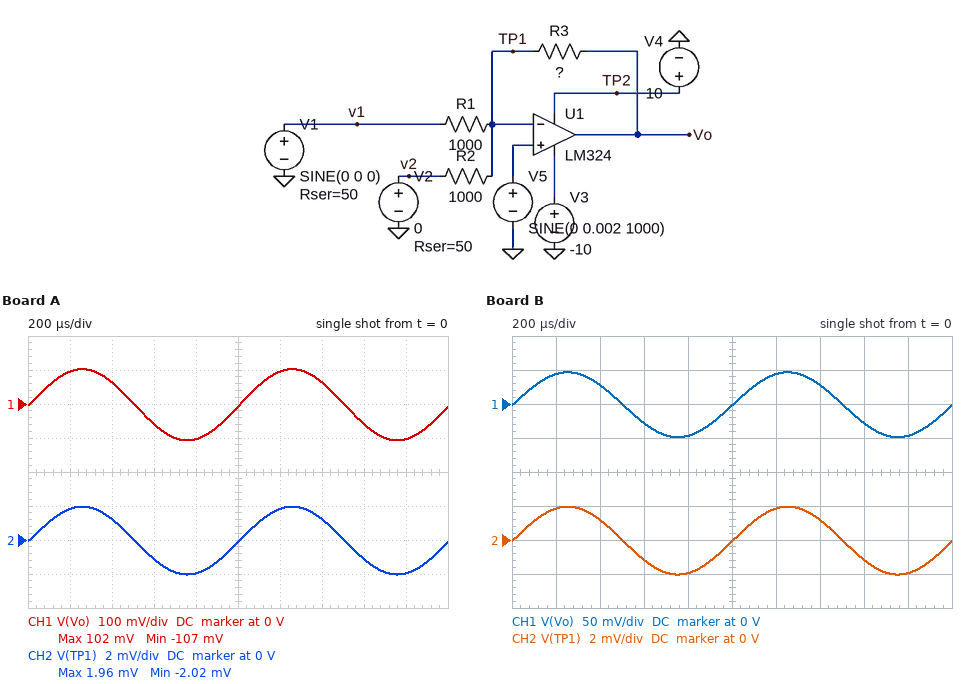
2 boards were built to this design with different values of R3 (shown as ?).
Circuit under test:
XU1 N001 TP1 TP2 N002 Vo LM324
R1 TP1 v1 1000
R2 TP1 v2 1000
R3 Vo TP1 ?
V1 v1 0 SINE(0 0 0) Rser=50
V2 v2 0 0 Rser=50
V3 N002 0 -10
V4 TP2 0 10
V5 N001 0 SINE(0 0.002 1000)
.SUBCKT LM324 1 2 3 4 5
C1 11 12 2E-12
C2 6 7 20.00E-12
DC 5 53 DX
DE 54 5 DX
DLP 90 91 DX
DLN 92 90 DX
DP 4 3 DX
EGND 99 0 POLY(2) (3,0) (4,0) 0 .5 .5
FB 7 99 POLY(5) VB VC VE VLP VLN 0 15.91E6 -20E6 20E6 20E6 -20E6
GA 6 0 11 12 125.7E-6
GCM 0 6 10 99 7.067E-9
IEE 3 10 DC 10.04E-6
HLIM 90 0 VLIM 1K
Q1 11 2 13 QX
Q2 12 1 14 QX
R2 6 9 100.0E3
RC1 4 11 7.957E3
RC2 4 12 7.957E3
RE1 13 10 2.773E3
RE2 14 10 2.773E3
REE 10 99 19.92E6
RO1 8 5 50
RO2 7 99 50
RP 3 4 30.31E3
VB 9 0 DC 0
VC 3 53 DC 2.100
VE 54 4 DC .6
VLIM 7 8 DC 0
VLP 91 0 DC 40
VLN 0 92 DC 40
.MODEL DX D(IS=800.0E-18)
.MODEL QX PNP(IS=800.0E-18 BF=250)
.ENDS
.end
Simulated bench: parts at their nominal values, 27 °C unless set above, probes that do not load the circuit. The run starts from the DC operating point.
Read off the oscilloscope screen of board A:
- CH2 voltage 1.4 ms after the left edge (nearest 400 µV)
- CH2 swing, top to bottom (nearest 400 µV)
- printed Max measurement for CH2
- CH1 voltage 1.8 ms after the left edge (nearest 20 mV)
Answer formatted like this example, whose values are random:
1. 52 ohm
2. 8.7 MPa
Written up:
1. 1.2 mV
2. 4.0 mV
3. 1.96 mV
4. -100 mV
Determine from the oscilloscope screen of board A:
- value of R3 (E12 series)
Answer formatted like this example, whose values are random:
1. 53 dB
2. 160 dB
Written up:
1. 27 kΩ
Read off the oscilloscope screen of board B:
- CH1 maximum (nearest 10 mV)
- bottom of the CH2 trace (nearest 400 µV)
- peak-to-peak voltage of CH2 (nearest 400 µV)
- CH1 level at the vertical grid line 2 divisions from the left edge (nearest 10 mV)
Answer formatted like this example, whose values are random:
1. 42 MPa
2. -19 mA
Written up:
1. 50 mV
2. -2.0 mV
3. 4.0 mV
4. 30 mV
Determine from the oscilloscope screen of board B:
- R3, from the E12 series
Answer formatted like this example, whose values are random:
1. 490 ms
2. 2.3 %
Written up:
1. 12 kΩ
